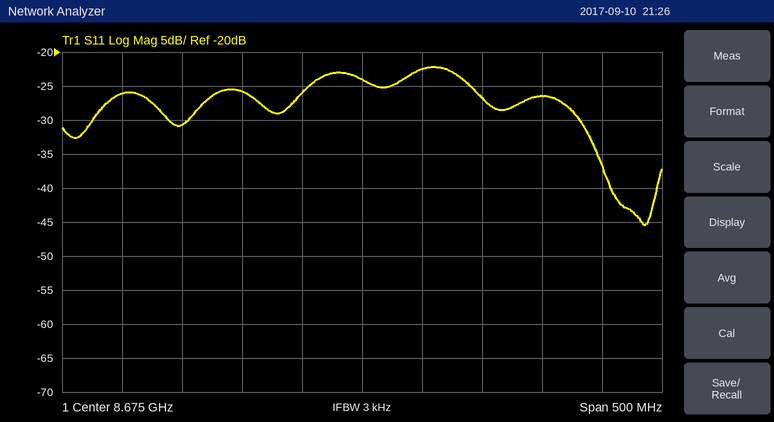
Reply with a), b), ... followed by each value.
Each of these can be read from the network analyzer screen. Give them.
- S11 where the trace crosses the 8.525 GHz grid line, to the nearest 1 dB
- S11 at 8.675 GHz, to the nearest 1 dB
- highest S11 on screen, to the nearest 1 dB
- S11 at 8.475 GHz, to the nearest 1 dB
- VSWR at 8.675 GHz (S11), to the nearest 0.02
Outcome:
a) -31 dB
b) -24 dB
c) -22 dB
d) -26 dB
e) 1.14
